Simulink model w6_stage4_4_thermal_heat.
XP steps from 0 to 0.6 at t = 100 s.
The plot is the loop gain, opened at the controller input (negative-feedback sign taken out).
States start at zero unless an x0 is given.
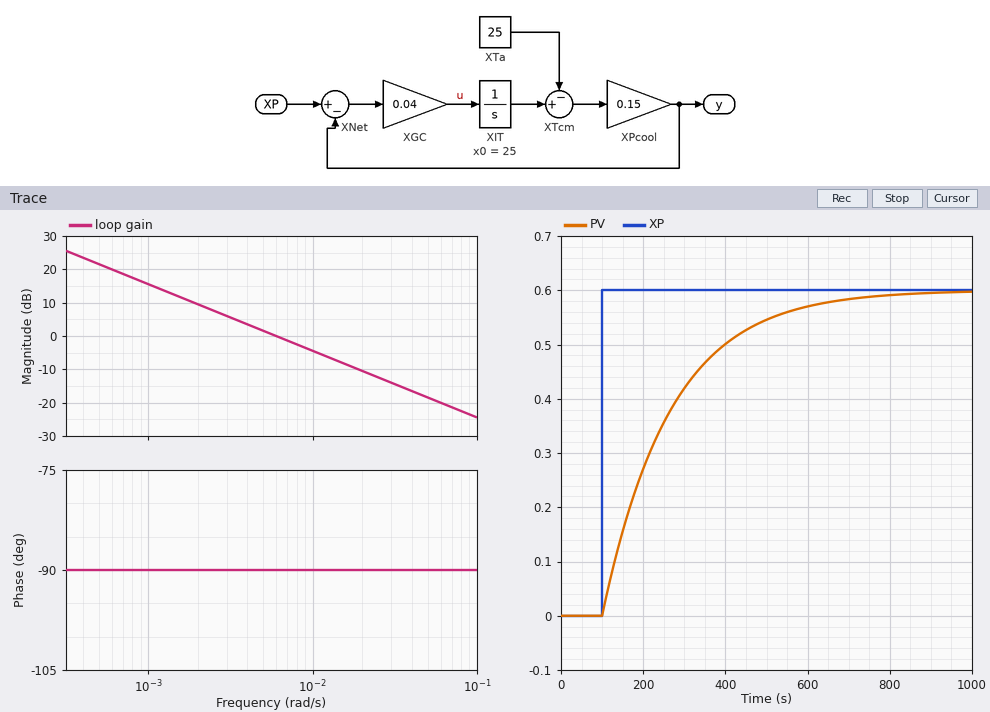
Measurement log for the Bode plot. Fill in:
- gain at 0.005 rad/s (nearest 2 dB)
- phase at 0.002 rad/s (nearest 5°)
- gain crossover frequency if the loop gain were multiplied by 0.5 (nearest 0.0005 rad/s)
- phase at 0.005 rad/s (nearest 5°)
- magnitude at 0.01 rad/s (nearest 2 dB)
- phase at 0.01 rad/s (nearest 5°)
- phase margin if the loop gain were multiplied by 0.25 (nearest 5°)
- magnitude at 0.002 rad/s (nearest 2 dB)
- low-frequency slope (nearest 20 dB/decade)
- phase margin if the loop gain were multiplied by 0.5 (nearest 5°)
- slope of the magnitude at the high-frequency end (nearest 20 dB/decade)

2 dB
-90°
0.0030 rad/s
-90°
-4 dB
-90°
90°
10 dB
-20 dB/decade
90°
-20 dB/decade
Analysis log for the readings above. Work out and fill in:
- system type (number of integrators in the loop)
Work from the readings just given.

1
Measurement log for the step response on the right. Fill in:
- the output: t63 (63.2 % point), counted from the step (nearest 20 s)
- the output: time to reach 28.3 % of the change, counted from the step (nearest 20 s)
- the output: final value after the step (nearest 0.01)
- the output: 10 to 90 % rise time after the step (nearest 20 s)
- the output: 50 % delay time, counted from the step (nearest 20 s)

160 s
60 s
0.60
360 s
120 s
